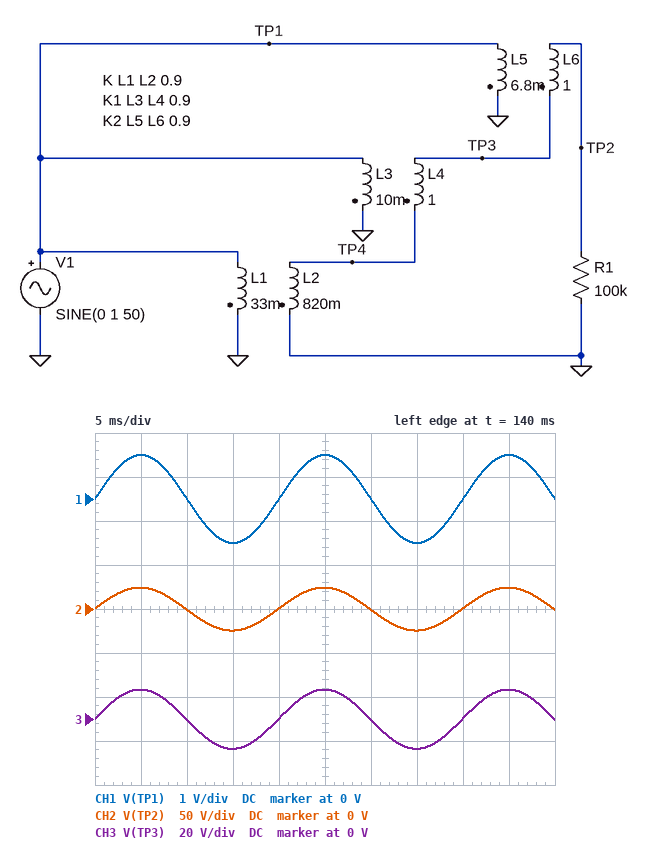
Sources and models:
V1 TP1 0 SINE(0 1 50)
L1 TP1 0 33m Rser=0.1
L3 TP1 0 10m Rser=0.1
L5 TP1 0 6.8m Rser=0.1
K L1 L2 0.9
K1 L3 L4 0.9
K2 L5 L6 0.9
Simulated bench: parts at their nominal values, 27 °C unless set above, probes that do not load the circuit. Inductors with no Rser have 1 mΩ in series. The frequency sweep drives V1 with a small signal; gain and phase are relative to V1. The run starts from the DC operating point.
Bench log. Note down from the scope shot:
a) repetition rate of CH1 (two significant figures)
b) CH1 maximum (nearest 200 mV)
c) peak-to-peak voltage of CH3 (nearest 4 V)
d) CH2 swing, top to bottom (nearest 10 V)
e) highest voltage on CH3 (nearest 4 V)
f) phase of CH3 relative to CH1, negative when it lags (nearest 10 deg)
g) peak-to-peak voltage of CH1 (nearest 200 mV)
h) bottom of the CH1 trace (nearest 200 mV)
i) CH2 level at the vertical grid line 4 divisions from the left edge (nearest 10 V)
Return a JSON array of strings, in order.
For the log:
["50 Hz", "1.0 V", "28 V", "50 V", "12 V", "0 deg", "2.0 V", "-1.0 V", "0 V"]
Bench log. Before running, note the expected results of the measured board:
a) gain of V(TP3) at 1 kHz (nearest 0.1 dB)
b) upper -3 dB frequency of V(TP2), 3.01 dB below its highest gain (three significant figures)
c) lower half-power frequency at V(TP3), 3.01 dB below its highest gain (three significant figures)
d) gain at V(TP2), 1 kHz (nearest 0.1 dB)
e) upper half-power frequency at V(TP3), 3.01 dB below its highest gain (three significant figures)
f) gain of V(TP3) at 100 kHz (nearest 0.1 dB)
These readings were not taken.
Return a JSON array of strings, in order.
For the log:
["22.6 dB", "29.7 kHz", "1.29 Hz", "27.7 dB", "30.6 kHz", "12.9 dB"]
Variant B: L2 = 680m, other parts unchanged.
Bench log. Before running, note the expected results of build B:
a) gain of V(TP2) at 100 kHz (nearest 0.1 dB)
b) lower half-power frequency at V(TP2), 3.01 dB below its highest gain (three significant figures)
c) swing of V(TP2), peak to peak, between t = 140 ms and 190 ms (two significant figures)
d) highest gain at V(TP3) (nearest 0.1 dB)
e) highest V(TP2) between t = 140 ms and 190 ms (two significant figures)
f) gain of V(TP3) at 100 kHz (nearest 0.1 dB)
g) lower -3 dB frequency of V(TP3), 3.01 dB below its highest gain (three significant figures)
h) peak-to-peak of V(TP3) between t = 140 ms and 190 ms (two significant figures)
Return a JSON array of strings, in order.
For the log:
["17.1 dB", "1.84 Hz", "48 V", "22.3 dB", "24 V", "12.7 dB", "1.32 Hz", "26 V"]
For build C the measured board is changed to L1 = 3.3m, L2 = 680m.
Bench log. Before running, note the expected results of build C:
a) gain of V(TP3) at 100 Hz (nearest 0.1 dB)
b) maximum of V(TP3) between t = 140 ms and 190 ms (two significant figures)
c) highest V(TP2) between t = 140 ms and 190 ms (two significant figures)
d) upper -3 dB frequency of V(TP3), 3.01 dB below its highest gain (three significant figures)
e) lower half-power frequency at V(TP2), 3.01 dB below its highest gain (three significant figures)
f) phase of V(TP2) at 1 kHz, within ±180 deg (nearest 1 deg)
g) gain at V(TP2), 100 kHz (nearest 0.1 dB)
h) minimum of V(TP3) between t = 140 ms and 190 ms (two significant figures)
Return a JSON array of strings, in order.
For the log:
["26.8 dB", "22 V", "33 V", "31.4 kHz", "3.11 Hz", "-2 deg", "19.8 dB", "-22 V"]
